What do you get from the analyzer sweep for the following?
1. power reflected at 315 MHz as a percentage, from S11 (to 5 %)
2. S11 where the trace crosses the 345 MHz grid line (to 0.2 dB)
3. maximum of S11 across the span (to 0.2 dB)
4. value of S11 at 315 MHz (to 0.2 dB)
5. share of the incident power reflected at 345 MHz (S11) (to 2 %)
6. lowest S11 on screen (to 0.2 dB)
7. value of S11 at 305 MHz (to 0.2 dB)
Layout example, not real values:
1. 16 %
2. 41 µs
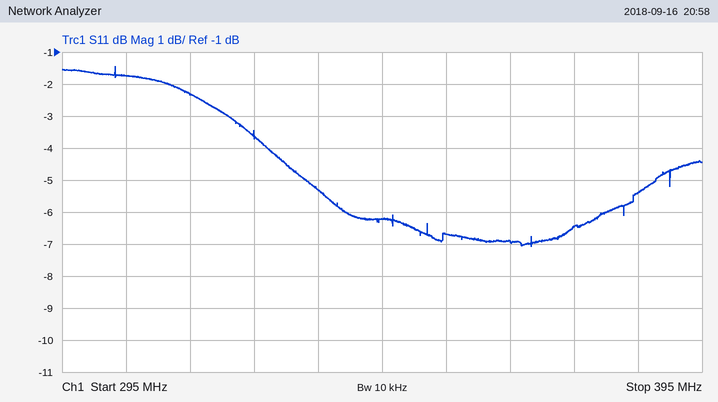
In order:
1. 60 %
2. -6.2 dB
3. -1.4 dB
4. -2.4 dB
5. 24 %
6. -7.0 dB
7. -1.8 dB
